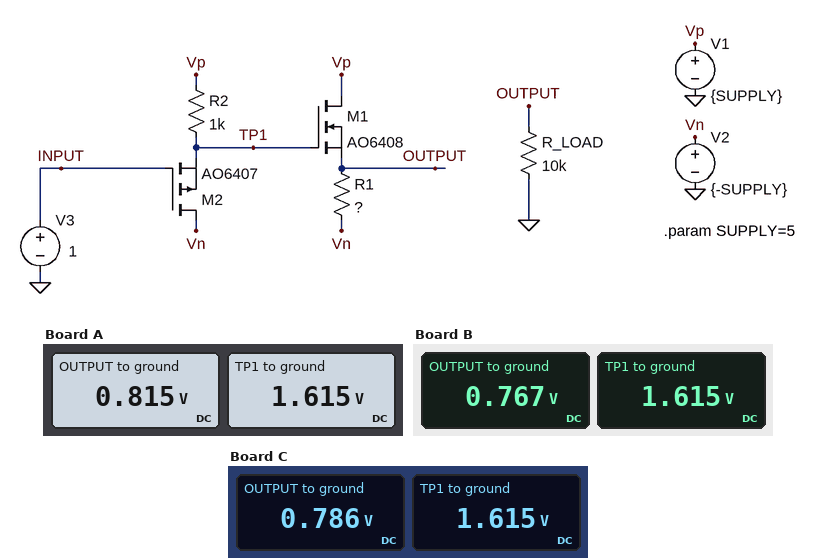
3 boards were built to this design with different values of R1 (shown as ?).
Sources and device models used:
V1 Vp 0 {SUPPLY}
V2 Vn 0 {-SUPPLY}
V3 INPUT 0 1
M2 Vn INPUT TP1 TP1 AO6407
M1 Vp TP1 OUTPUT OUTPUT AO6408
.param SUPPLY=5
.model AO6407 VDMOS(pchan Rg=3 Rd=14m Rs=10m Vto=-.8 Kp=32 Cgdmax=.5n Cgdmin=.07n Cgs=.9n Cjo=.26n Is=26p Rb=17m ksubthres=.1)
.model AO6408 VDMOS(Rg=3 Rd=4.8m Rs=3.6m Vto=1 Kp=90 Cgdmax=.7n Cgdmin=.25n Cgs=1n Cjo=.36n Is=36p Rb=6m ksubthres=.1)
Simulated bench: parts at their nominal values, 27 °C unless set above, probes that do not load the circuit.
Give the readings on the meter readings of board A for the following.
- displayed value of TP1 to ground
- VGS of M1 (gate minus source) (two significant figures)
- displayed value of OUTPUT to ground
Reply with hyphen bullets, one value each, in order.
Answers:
- 1.615 V
- 800 mV
- 0.815 V
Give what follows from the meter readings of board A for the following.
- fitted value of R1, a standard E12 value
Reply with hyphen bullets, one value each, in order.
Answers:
- 820 Ω
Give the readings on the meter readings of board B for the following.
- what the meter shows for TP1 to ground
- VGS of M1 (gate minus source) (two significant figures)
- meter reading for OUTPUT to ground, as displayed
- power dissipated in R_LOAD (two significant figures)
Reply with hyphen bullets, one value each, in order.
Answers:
- 1.615 V
- 850 mV
- 0.767 V
- 59 µW
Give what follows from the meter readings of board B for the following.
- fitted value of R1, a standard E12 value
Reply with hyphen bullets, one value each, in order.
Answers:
- 330 Ω
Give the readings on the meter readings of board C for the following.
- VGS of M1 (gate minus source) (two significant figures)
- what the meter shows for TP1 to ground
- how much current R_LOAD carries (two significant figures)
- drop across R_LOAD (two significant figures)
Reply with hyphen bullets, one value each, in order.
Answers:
- 830 mV
- 1.615 V
- 79 µA
- 790 mV
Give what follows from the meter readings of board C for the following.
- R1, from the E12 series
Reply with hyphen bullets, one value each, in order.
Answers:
- 470 Ω
